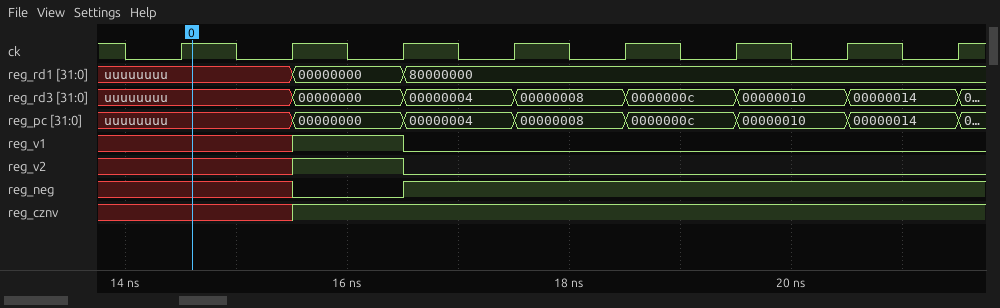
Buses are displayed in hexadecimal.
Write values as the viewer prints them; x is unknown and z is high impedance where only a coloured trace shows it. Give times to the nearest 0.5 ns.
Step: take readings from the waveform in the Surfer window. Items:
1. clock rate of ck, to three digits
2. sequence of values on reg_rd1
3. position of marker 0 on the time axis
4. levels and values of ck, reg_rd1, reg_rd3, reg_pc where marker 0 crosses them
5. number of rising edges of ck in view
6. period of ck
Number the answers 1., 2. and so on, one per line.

1. 1.00 GHz
2. uuuuuuuu, 00000000, 80000000
3. 14.5 ns
4. ck=1, reg_rd1=uuuuuuuu, reg_rd3=uuuuuuuu, reg_pc=uuuuuuuu
5. 8
6. 1 ns
